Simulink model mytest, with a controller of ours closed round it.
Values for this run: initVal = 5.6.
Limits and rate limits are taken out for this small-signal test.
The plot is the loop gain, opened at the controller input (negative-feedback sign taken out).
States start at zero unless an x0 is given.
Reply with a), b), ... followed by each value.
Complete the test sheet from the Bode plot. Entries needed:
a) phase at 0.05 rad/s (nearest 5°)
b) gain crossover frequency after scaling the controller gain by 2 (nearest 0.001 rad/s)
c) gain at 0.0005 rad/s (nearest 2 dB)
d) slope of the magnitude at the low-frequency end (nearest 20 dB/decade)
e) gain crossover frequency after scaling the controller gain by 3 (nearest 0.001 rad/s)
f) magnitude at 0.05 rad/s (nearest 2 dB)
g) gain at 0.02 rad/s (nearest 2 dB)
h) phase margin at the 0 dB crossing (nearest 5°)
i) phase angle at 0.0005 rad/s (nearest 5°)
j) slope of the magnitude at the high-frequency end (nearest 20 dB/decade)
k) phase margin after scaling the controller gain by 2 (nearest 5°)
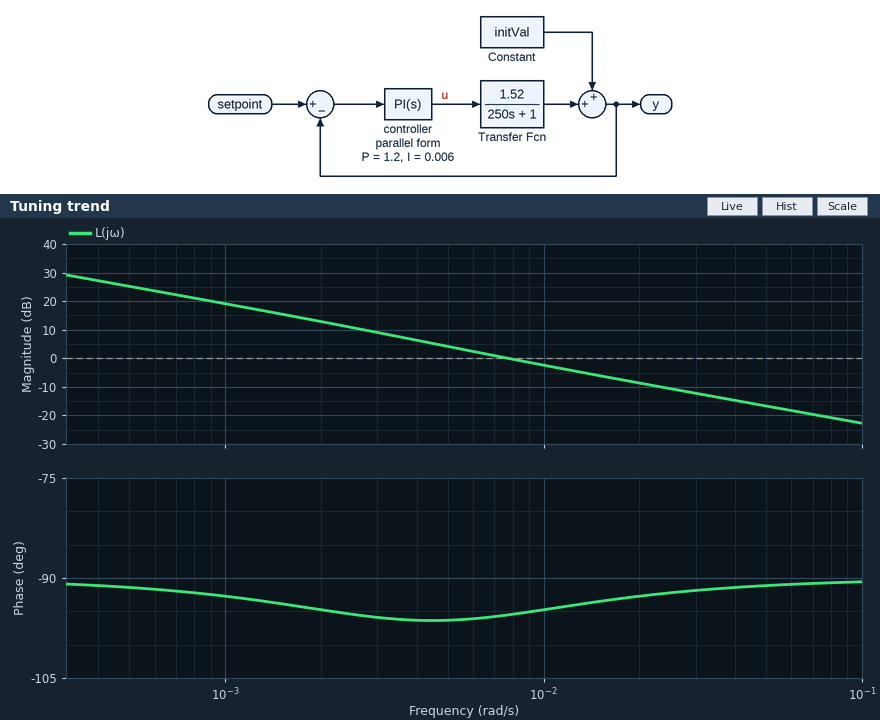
a) -90°
b) 0.015 rad/s
c) 26 dB
d) -20 dB/decade
e) 0.022 rad/s
f) -16 dB
g) -8 dB
h) 85°
i) -90°
j) -20 dB/decade
k) 85°
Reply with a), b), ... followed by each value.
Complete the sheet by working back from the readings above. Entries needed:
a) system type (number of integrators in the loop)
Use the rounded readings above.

a) 1
